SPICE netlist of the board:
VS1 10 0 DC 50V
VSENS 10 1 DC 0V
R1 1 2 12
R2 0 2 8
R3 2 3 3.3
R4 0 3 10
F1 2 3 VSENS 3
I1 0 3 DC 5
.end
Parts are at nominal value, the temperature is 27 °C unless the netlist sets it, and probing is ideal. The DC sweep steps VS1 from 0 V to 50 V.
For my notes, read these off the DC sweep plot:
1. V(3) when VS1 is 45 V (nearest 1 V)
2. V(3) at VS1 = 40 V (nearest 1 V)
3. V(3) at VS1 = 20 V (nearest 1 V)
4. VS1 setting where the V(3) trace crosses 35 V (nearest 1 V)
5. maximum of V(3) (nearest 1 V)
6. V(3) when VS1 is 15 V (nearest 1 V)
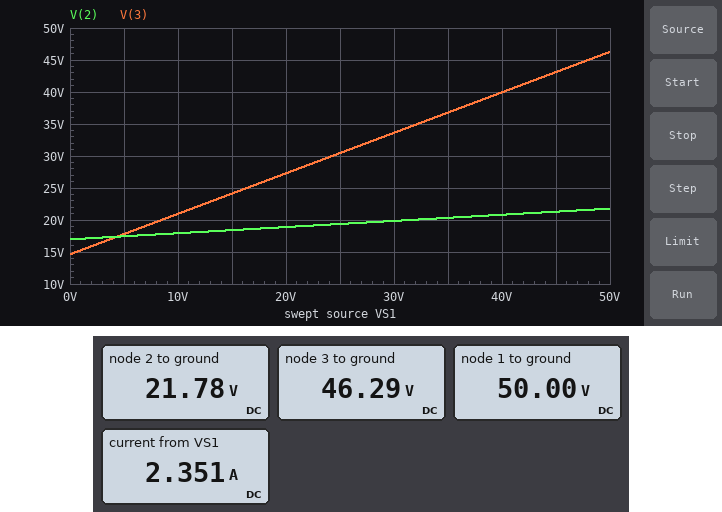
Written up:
43 V
40 V
27 V
32 V
46 V
24 V
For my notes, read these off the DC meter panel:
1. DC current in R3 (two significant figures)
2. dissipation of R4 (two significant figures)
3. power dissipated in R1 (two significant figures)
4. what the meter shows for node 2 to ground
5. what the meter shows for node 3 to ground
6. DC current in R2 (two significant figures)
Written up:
7.4 A
210 W
66 W
21.78 V
46.29 V
2.7 A
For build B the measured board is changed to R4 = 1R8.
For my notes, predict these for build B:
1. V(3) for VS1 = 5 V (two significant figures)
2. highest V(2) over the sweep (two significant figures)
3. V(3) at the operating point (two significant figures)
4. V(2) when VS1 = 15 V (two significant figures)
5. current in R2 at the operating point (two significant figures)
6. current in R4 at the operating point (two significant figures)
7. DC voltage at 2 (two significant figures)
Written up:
7.6 V
7.3 V
20 V
2.4 V
1.1 A
11 A
-8.9 V
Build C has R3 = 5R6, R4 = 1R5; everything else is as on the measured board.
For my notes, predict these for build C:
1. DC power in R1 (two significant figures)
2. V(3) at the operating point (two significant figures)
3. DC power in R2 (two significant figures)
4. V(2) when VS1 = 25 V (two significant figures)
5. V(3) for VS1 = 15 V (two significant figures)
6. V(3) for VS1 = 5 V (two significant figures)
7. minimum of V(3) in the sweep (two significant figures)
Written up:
540 W
23 V
120 W
-12 V
11 V
7.1 V
5.3 V
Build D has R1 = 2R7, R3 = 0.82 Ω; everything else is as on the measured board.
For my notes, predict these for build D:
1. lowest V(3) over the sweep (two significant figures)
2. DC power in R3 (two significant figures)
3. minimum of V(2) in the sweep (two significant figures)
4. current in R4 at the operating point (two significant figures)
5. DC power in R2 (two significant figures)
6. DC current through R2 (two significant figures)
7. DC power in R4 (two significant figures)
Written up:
4.5 V
160 W
9.2 V
4.9 A
180 W
4.7 A
240 W
